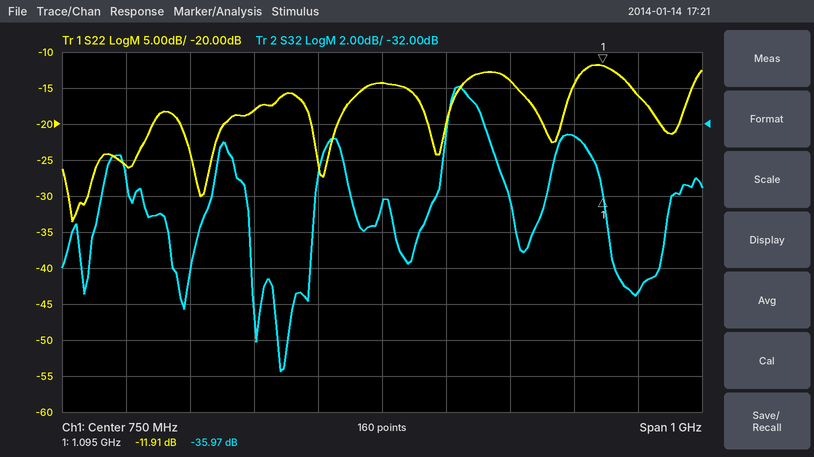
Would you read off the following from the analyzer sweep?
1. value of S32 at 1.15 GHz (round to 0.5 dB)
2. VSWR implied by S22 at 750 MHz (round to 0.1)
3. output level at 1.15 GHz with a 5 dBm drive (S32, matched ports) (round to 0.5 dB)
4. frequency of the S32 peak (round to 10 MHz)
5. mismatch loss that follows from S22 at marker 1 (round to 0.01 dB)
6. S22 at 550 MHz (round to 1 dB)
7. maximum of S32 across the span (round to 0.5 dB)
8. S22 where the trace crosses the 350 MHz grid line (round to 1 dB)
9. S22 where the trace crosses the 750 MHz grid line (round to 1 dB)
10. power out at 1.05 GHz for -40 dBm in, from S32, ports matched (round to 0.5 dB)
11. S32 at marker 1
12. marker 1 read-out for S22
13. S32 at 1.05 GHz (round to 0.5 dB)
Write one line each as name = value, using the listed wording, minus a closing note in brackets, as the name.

value of S32 at 1.15 GHz = -41.5 dB
VSWR implied by S22 at 750 MHz = 1.5
output level at 1.15 GHz with a 5 dBm drive (S32, matched ports) = -36.5 dBm
frequency of the S32 peak = 870 MHz
mismatch loss that follows from S22 at marker 1 = 0.29 dB
S22 at 550 MHz = -18 dB
maximum of S32 across the span = -30.0 dB
S22 where the trace crosses the 350 MHz grid line = -26 dB
S22 where the trace crosses the 750 MHz grid line = -14 dB
power out at 1.05 GHz for -40 dBm in, from S32, ports matched = -72.5 dBm
S32 at marker 1 = -35.97 dB
marker 1 read-out for S22 = -11.91 dB
S32 at 1.05 GHz = -32.5 dB
